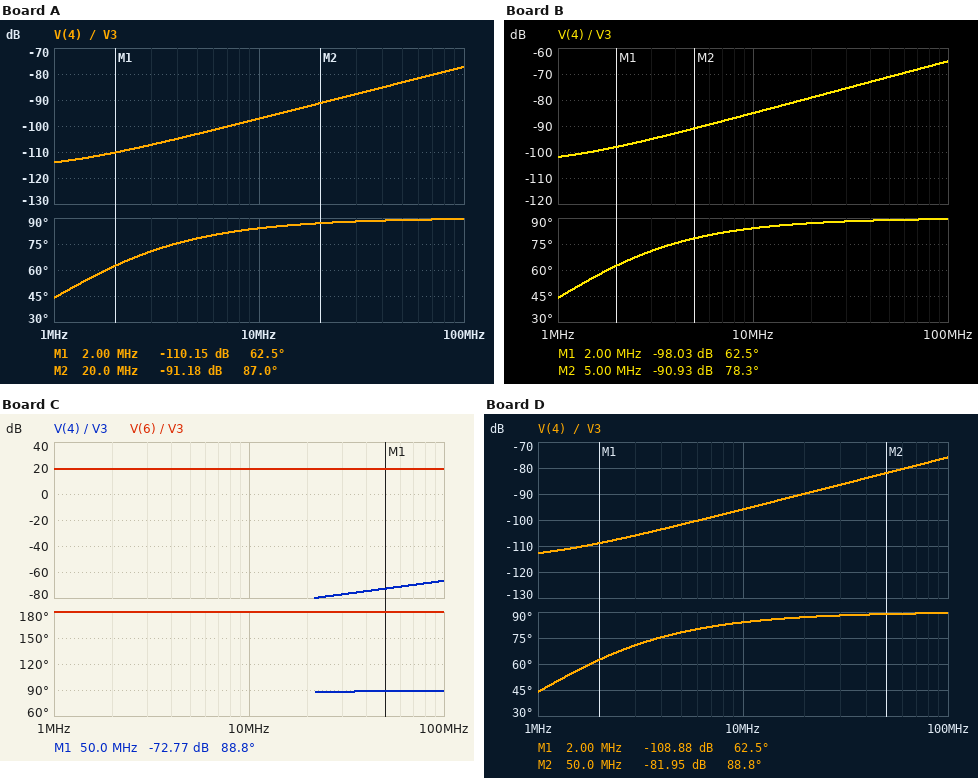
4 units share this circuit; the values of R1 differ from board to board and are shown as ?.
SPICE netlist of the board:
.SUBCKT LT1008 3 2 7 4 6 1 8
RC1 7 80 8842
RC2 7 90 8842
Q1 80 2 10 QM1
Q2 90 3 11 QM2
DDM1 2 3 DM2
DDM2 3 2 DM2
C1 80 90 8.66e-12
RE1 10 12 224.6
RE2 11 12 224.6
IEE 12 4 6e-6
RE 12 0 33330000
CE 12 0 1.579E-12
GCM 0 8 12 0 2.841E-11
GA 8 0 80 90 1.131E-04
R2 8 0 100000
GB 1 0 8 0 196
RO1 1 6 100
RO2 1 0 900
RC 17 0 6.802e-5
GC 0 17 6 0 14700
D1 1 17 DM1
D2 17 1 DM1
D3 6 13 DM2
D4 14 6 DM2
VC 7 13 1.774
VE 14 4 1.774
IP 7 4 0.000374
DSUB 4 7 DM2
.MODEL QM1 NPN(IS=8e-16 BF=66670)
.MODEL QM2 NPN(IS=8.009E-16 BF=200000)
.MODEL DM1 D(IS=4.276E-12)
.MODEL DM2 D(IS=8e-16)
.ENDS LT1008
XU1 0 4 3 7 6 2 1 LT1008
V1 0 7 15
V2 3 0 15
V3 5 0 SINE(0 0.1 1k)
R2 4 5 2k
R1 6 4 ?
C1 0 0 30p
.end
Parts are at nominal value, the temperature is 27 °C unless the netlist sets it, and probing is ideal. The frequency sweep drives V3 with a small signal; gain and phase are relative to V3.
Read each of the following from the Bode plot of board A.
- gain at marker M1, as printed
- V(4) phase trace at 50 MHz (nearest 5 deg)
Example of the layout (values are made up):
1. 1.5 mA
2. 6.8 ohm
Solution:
1. -110.15 dB
2. 90 deg
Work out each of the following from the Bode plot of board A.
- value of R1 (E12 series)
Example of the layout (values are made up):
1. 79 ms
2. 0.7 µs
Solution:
1. 4.7 kΩ
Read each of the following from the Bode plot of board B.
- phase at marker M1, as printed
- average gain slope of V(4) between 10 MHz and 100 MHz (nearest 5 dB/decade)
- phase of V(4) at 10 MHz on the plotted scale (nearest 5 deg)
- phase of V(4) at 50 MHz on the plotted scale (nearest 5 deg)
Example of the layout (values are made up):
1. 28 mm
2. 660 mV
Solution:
1. 62.5 deg
2. 20 dB/decade
3. 85 deg
4. 90 deg
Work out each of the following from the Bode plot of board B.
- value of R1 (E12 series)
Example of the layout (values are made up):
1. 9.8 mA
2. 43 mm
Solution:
1. 22 kΩ
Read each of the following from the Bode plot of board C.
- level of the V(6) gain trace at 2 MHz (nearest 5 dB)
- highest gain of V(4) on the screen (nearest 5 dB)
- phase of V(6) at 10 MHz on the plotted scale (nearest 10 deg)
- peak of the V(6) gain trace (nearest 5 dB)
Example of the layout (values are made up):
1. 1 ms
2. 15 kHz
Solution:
1. 20 dB
2. -65 dB
3. 180 deg
4. 20 dB
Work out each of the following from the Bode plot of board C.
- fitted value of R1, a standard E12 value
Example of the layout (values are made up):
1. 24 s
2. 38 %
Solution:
1. 18 kΩ
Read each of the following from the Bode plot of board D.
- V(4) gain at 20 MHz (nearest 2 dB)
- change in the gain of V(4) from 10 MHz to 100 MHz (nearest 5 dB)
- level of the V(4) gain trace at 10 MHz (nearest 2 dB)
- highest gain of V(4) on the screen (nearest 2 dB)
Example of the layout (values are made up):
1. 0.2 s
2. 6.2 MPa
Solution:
1. -90 dB
2. 20 dB
3. -96 dB
4. -76 dB
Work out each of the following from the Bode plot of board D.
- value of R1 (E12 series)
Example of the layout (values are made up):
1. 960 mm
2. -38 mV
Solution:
1. 5.6 kΩ
